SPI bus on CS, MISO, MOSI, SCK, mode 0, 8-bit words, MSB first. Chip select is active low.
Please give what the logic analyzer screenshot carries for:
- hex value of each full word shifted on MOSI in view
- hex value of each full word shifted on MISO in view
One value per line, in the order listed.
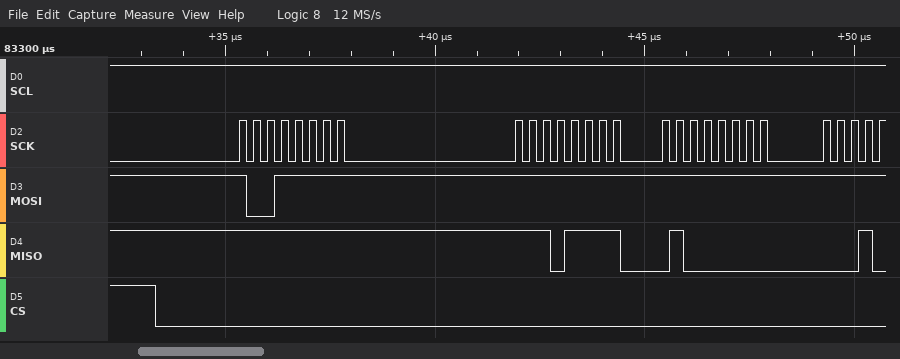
9F, FF, FF
FF, EF, 40
